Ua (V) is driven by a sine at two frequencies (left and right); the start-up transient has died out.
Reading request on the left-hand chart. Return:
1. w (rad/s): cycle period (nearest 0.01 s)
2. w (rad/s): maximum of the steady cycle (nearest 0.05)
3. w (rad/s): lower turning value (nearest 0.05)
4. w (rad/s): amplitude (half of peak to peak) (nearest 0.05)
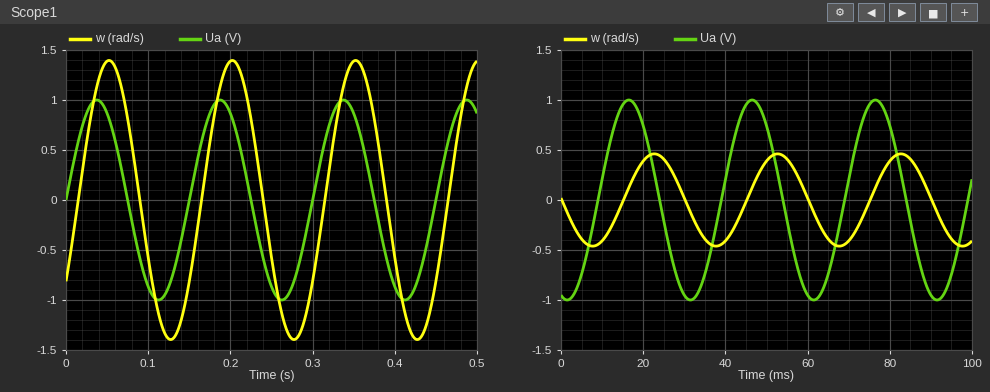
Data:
0.15 s
1.40
-1.40
1.40
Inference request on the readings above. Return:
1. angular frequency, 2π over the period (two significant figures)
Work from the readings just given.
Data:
42 rad/s
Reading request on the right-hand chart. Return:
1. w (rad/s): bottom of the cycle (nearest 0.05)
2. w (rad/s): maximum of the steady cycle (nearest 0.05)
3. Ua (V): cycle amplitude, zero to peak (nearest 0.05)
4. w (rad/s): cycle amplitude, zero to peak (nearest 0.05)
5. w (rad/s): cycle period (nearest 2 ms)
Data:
-0.45
0.45
1.00
0.45
30 ms
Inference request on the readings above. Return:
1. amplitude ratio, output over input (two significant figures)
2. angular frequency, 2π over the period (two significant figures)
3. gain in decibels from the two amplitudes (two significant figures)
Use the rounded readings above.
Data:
0.45
0.21 rad/ms
-6.9 dB
